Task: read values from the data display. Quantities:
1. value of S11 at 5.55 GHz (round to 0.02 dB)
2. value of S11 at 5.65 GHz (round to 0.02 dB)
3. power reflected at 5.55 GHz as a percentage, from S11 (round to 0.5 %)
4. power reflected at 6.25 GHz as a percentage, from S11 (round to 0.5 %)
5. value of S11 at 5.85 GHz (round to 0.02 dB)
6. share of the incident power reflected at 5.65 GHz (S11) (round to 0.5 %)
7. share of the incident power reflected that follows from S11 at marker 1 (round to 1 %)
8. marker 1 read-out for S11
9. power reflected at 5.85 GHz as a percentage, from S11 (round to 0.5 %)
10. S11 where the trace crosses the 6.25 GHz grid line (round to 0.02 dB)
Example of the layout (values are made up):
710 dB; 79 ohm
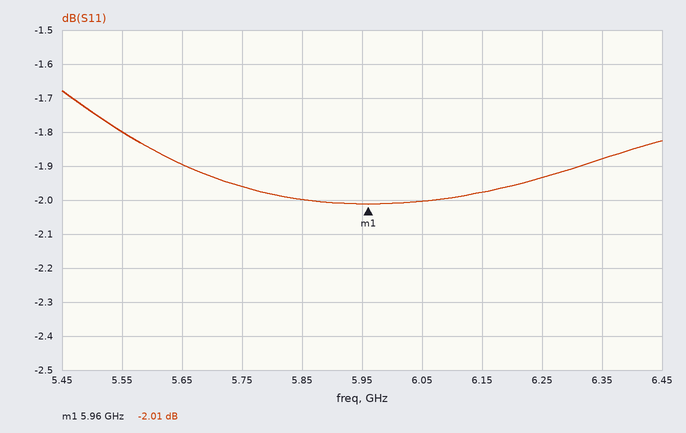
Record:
-1.80 dB; -1.90 dB; 66.0 %; 64.0 %; -2.00 dB; 64.5 %; 63 %; -2.01 dB; 63.0 %; -1.94 dB
